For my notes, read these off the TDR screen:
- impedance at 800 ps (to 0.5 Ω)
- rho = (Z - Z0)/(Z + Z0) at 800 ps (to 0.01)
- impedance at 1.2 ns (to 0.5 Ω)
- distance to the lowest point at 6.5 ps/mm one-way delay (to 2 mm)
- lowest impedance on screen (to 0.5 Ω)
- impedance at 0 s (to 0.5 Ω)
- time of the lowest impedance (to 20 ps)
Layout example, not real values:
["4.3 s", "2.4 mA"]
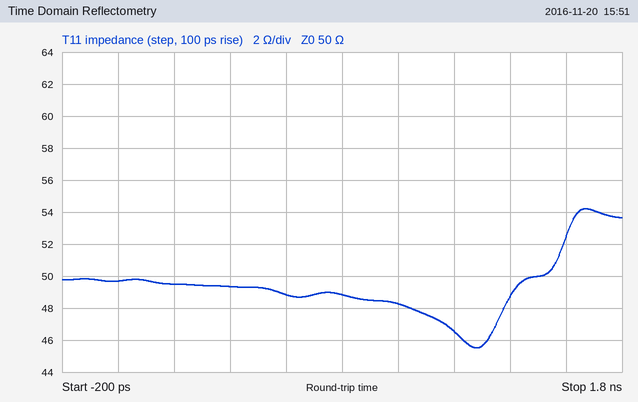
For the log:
["49.0 Ω", "-0.01", "46.5 Ω", "98 mm", "45.5 Ω", "49.5 Ω", "1.28 ns"]
